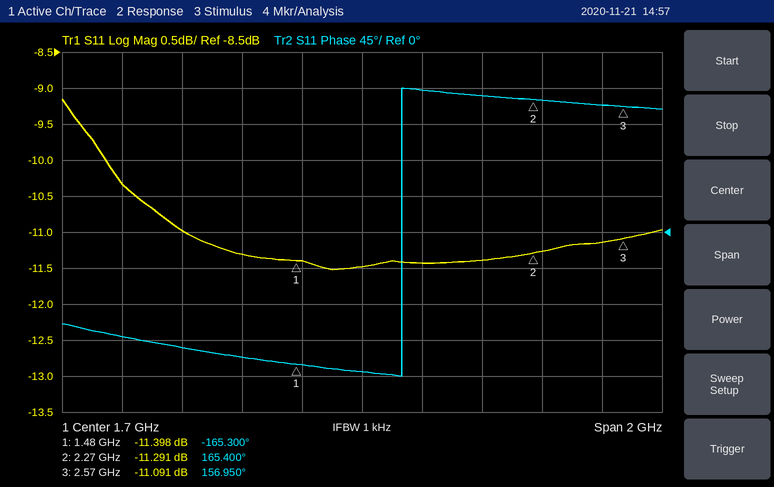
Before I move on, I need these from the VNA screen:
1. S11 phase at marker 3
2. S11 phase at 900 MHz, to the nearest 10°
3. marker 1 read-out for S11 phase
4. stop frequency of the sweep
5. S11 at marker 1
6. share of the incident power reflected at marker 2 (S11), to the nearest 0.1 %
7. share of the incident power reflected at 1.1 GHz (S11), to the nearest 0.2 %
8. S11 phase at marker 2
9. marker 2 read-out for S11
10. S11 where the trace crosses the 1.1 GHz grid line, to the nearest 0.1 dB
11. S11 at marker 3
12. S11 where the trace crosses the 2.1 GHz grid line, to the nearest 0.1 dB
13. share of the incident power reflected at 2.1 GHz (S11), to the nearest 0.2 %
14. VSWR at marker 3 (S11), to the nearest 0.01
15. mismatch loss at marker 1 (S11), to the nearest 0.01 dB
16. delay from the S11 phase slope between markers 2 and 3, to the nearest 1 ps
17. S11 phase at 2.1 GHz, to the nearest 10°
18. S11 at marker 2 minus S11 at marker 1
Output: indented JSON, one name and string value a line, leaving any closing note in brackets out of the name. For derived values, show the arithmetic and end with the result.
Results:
{
  "S11 phase at marker 3": "156.950°",
  "S11 phase at 900 MHz, to the nearest 10°": "-130°",
  "marker 1 read-out for S11 phase": "-165.300°",
  "stop frequency of the sweep": "2.7 GHz",
  "S11 at marker 1": "-11.398 dB",
  "share of the incident power reflected at marker 2 (S11), to the nearest 0.1 %": "10^(-11.291/10) ≈ 7.4 %",
  "share of the incident power reflected at 1.1 GHz (S11), to the nearest 0.2 %": "10^(-11/10) ≈ 7.94 %, so 8.0 % to the nearest 0.2 %",
  "S11 phase at marker 2": "165.400°",
  "marker 2 read-out for S11": "-11.291 dB",
  "S11 where the trace crosses the 1.1 GHz grid line, to the nearest 0.1 dB": "-11.0 dB",
  "S11 at marker 3": "-11.091 dB",
  "S11 where the trace crosses the 2.1 GHz grid line, to the nearest 0.1 dB": "-11.4 dB",
  "share of the incident power reflected at 2.1 GHz (S11), to the nearest 0.2 %": "10^(-11.4/10) ≈ 7.2 %",
  "VSWR at marker 3 (S11), to the nearest 0.01": "(1 + 0.2789)/(1 − 0.2789) ≈ 1.77",
  "mismatch loss at marker 1 (S11), to the nearest 0.01 dB": "−10 log10(1 − 10^(-11.398/10)) ≈ 0.33 dB",
  "delay from the S11 phase slope between markers 2 and 3, to the nearest 1 ps": "−(156.95° − (165.4°))/(360° × 300 MHz) ≈ 78 ps",
  "S11 phase at 2.1 GHz, to the nearest 10°": "170°",
  "S11 at marker 2 minus S11 at marker 1": "-11.291 − (-11.398) = 0.107 dB"
}
